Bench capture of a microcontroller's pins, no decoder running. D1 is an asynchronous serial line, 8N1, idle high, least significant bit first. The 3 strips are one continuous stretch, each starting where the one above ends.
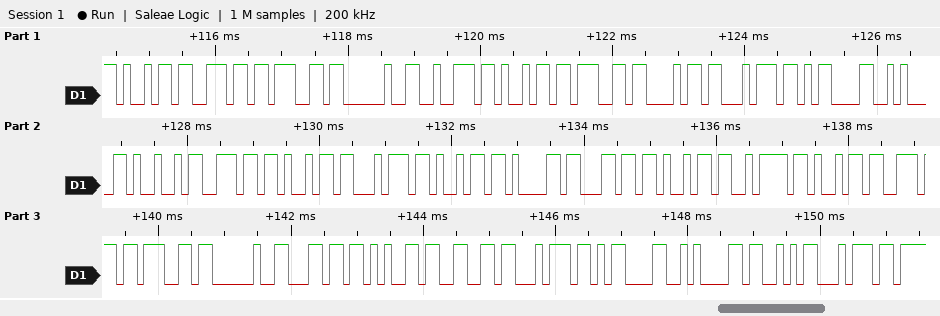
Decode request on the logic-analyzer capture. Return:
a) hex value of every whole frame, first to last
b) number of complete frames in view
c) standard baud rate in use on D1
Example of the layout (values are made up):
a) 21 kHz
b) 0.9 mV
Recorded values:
a) 69 6E 67 20 72 69 67 68 74 0D 0A 49 6E 69 74 69 61 6C 69 7A 69 6E 67 20 6C 65 66 74 0D 0A 53 74
b) 32
c) 9600 baud
